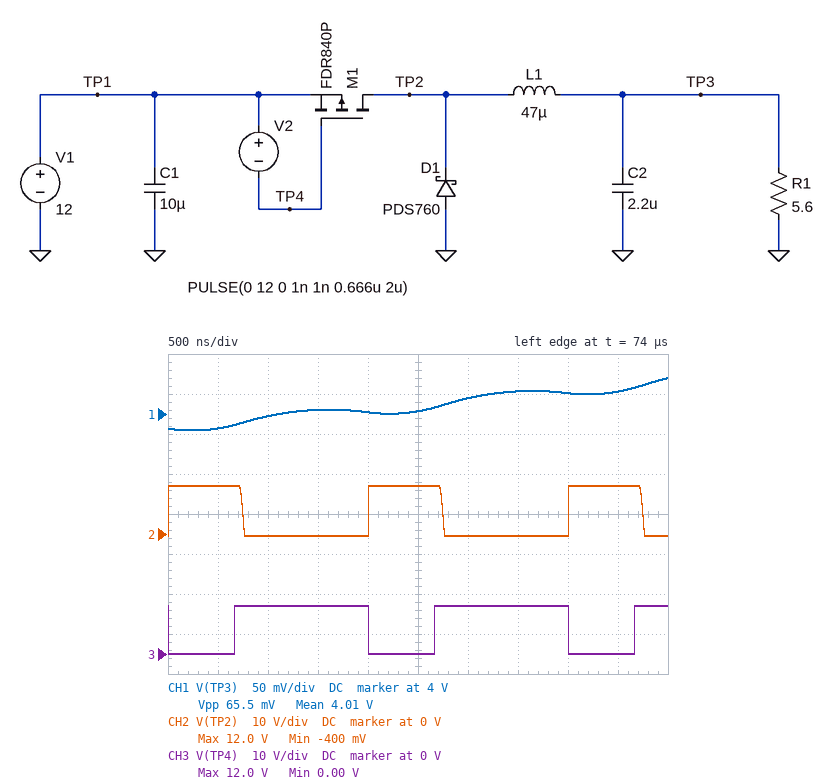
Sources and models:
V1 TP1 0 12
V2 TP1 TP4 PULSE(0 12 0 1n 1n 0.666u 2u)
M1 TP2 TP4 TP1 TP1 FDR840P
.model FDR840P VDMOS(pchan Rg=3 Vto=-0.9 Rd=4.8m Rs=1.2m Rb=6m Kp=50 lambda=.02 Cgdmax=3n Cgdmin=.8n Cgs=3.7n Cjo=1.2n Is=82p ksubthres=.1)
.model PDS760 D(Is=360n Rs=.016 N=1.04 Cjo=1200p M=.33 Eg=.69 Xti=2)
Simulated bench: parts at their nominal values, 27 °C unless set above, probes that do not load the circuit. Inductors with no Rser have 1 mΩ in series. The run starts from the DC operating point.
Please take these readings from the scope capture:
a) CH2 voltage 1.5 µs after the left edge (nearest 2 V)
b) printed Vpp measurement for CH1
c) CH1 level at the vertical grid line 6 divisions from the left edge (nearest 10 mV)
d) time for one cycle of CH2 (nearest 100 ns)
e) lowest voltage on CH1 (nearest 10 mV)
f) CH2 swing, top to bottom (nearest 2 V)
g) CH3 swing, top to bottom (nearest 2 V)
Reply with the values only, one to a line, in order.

0 V
65.5 mV
4.02 V
2.0 µs
3.98 V
12 V
12 V
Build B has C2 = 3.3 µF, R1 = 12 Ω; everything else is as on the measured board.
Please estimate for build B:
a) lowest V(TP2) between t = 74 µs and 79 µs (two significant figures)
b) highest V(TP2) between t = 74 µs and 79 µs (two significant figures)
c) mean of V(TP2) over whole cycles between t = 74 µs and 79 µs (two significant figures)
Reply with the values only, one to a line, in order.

-410 mV
12 V
4.4 V
